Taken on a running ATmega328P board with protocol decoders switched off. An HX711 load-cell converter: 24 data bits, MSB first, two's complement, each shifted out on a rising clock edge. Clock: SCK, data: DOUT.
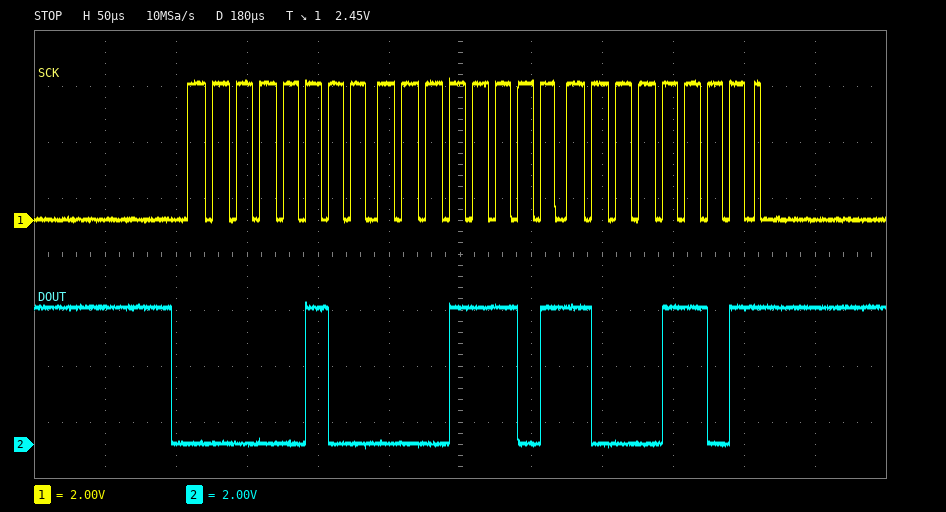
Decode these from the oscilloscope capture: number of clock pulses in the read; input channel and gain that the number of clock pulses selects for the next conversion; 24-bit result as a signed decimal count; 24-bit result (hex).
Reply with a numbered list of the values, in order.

1. 25
2. channel A, gain 128
3. 269709
4. 0x041D8D
